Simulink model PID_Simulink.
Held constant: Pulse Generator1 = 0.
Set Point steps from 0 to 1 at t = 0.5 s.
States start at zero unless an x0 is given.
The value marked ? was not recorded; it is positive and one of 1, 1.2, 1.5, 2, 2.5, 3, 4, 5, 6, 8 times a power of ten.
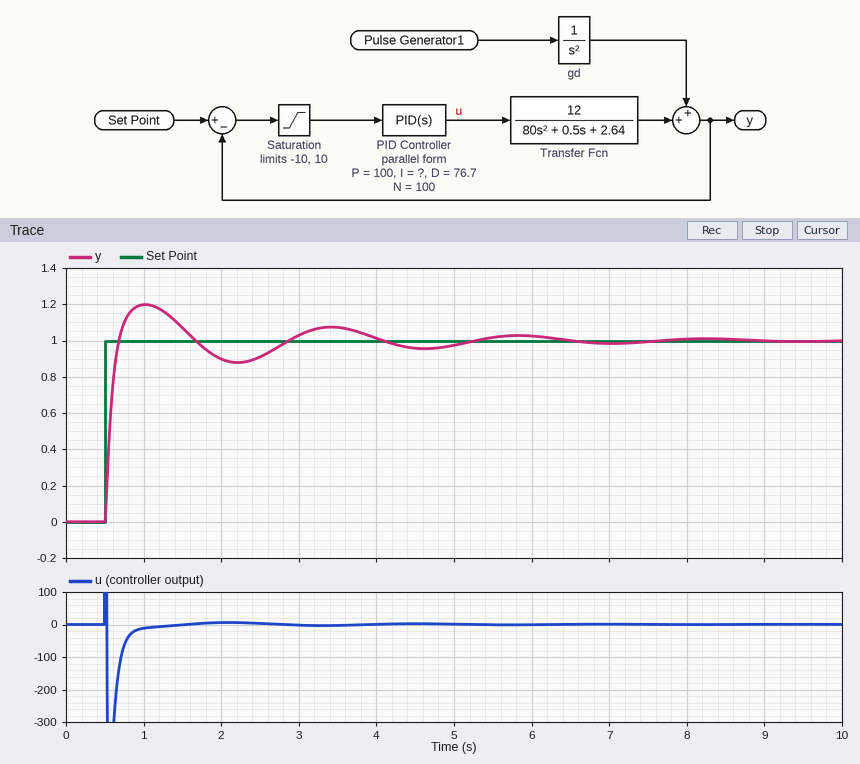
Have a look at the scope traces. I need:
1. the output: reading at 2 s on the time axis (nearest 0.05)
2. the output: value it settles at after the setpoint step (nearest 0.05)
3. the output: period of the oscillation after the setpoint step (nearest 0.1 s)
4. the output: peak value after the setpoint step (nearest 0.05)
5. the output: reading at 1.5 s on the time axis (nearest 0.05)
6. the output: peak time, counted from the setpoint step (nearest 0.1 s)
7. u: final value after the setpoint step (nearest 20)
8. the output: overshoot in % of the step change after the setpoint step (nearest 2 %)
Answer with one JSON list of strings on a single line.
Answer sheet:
["0.90", "1.00", "2.4 s", "1.20", "1.05", "0.5 s", "0", "20 %"]
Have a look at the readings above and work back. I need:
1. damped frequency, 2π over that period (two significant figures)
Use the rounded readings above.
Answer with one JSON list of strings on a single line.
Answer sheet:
["2.6 rad/s"]
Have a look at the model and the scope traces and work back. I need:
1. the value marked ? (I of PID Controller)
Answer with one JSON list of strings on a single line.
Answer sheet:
["500"]
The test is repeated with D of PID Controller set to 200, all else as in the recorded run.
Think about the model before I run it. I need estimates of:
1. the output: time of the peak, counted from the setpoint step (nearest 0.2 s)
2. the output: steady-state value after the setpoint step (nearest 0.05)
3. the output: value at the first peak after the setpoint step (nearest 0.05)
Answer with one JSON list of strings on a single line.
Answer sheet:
["0.8 s", "1.00", "1.05"]
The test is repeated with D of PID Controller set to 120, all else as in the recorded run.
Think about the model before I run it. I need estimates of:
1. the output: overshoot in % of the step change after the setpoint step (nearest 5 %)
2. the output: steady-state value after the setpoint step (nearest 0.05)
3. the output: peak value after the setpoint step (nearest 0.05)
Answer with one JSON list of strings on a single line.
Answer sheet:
["10 %", "1.00", "1.10"]
